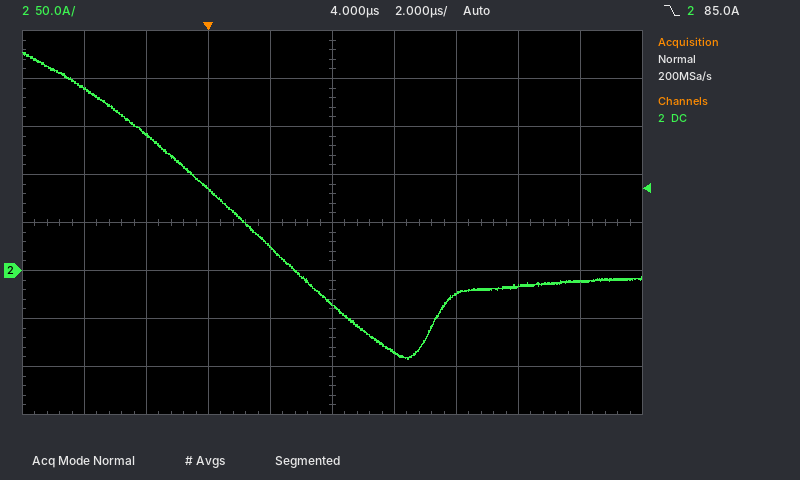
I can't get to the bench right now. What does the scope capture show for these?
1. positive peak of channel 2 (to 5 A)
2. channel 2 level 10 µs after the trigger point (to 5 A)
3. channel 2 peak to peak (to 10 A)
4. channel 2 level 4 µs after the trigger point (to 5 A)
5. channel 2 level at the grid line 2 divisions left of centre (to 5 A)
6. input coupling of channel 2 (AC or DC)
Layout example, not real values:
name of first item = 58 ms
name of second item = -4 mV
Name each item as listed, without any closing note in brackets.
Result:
positive peak of channel 2 = 225 A
channel 2 level 10 µs after the trigger point = -15 A
channel 2 peak to peak = 320 A
channel 2 level 4 µs after the trigger point = -35 A
channel 2 level at the grid line 2 divisions left of centre = 85 A
input coupling of channel 2 = DC
